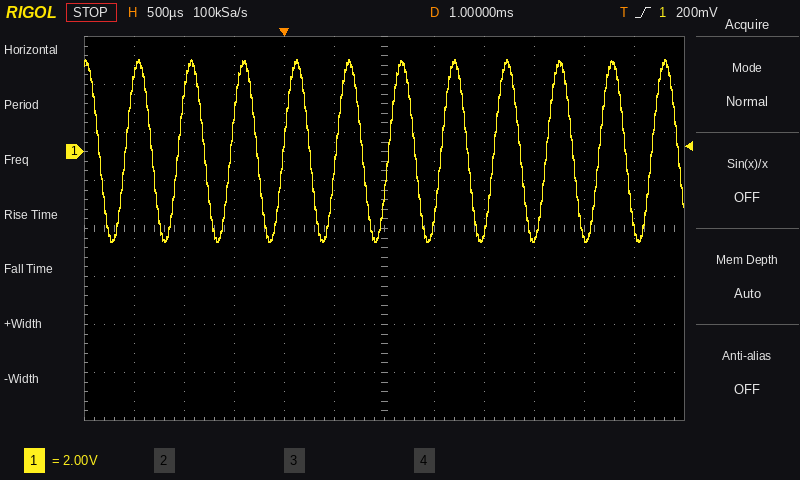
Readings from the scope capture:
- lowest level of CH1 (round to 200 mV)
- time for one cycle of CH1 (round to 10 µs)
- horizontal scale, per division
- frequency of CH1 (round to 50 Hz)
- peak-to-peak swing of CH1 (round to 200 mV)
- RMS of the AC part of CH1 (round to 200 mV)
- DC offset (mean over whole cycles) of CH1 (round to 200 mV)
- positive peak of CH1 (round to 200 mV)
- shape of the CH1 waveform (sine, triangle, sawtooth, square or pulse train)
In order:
-3.8 V
530 µs
500 µs
1.90 kHz
7.6 V
2.6 V
0.0 V
3.8 V
sine
